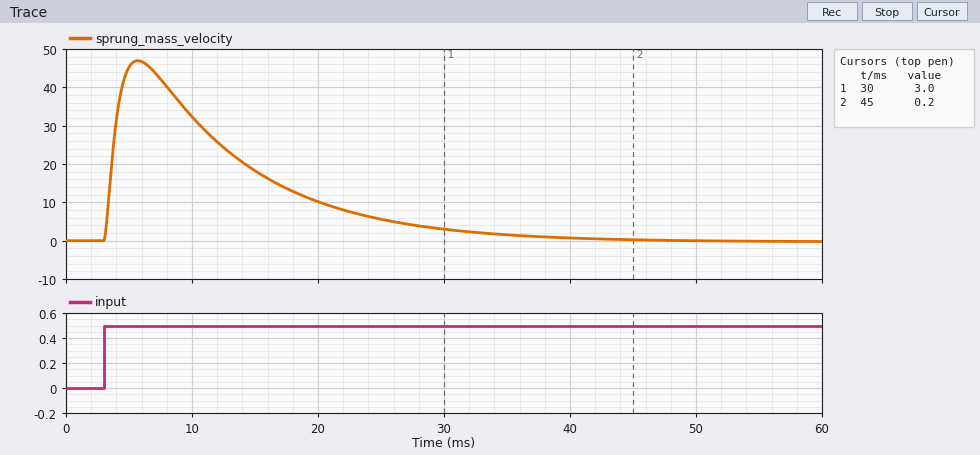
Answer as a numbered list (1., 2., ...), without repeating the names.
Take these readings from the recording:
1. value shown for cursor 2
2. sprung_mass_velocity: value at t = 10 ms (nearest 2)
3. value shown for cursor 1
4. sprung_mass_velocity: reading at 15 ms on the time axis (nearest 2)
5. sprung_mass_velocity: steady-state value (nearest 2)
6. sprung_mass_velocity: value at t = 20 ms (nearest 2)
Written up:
1. 0.2
2. 32
3. 3.0
4. 18
5. 0
6. 10
